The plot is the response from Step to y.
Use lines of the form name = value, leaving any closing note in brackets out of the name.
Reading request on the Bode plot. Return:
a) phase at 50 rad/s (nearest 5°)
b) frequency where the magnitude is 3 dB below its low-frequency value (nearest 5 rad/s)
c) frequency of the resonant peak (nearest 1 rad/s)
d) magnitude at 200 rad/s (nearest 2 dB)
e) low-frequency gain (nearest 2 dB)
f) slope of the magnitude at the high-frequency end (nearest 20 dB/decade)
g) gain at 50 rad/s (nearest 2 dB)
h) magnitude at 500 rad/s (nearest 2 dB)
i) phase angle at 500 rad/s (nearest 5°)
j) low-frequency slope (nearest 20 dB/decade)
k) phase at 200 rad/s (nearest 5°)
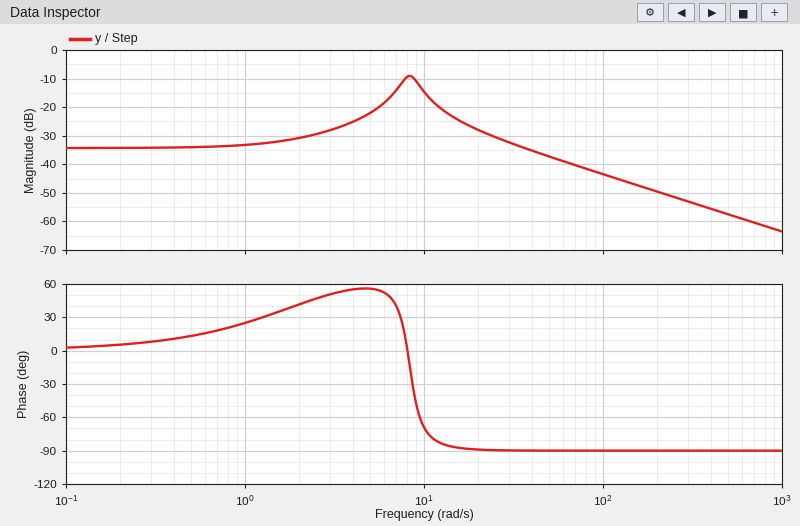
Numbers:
phase at 50 rad/s = -90°
frequency where the magnitude is 3 dB below its low-frequency value = 50 rad/s
frequency of the resonant peak = 8 rad/s
magnitude at 200 rad/s = -50 dB
low-frequency gain = -34 dB
slope of the magnitude at the high-frequency end = -20 dB/decade
gain at 50 rad/s = -38 dB
magnitude at 500 rad/s = -58 dB
phase angle at 500 rad/s = -90°
low-frequency slope = 0 dB/decade
phase at 200 rad/s = -90°
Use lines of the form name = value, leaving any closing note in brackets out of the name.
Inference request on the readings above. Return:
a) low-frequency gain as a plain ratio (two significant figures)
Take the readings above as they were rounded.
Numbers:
low-frequency gain as a plain ratio = 0.020
